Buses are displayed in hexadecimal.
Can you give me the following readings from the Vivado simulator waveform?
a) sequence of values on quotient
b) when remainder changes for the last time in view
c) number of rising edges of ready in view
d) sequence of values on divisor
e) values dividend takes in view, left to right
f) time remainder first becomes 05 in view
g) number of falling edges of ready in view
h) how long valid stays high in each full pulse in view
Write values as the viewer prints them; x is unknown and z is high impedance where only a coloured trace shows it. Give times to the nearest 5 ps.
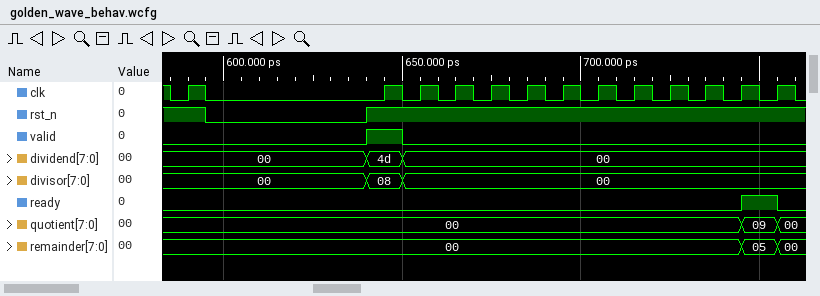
00, 09, 00
755 ps
1
00, 08, 00
00, 4d, 00
745 ps
1
10 ps
